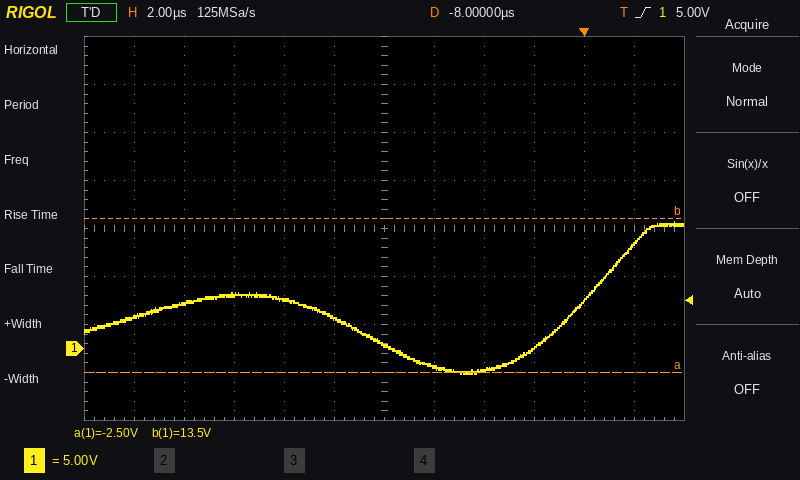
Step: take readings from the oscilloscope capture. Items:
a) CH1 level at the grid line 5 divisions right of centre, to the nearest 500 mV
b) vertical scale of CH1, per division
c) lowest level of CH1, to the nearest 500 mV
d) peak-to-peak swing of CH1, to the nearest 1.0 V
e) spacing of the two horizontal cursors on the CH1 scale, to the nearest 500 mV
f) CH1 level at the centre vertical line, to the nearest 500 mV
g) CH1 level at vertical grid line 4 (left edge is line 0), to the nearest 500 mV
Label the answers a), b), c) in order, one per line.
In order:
a) 11.0 V
b) 5 V
c) -2.5 V
d) 16.0 V
e) 16.0 V
f) 500 mV
g) 5.0 V
